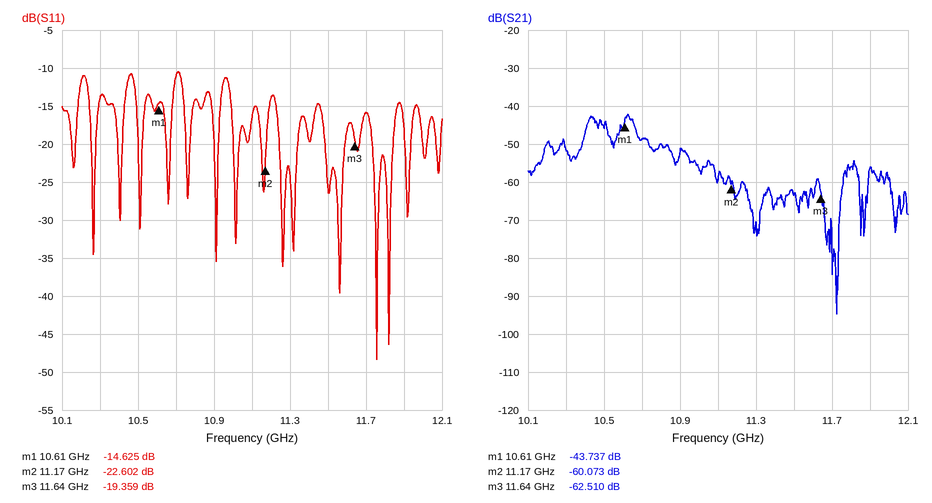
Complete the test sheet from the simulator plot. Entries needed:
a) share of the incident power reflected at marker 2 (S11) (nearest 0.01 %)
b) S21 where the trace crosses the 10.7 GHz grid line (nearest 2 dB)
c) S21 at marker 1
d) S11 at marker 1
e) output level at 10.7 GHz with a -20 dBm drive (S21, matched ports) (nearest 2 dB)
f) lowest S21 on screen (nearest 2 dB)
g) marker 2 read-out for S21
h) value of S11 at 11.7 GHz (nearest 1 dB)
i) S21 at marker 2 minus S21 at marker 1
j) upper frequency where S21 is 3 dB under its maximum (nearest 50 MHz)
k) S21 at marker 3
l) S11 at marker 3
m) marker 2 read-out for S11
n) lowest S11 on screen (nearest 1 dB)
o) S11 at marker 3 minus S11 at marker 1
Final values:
0.55 %
-48 dB
-43.737 dB
-14.625 dB
-68 dBm
-94 dB
-60.073 dB
-16 dB
-16.336 dB
10.65 GHz
-62.510 dB
-19.359 dB
-22.602 dB
-48 dB
-4.734 dB
